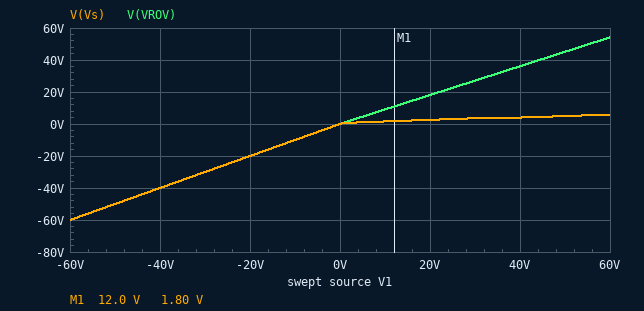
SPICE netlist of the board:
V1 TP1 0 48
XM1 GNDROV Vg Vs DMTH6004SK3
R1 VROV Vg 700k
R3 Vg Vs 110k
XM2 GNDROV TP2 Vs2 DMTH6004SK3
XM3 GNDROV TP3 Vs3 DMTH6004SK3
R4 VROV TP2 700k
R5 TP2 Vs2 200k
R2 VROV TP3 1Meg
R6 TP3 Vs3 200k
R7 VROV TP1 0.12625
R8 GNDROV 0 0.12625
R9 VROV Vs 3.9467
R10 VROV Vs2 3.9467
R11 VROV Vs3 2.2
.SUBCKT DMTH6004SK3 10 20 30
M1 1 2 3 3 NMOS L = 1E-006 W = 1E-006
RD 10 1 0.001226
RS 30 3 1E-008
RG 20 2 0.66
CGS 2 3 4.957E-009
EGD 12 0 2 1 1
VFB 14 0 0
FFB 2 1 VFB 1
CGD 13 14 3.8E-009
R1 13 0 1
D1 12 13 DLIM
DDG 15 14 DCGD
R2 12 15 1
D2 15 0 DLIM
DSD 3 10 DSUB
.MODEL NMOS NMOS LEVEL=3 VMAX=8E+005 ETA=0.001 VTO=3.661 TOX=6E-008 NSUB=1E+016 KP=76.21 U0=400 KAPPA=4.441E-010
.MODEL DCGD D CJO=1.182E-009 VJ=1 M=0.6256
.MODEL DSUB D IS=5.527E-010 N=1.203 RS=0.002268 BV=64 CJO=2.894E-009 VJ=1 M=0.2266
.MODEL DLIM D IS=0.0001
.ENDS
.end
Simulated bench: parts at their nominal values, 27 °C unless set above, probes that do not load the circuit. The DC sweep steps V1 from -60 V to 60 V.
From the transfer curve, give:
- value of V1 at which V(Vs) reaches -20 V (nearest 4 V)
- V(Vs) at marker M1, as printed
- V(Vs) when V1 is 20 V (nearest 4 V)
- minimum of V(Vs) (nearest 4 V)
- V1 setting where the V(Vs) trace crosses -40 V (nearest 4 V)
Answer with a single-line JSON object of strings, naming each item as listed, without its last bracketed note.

{"value of V1 at which V(Vs) reaches -20 V": "-20 V", "V(Vs) at marker M1, as printed": "1.80 V", "V(Vs) when V1 is 20 V": "4 V", "minimum of V(Vs)": "-60 V", "V1 setting where the V(Vs) trace crosses -40 V": "-40 V"}
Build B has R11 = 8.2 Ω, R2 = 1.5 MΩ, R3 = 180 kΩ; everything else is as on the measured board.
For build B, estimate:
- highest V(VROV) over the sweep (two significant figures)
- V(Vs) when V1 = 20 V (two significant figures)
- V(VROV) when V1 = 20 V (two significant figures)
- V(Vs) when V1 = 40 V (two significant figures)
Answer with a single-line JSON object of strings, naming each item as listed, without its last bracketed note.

{"highest V(VROV) over the sweep": "56 V", "V(Vs) when V1 = 20 V": "1.8 V", "V(VROV) when V1 = 20 V": "19 V", "V(Vs) when V1 = 40 V": "2.8 V"}
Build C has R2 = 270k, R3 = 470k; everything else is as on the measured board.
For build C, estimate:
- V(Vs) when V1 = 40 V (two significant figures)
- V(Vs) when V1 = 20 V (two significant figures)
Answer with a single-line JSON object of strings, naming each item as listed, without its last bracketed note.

{"V(Vs) when V1 = 40 V": "3.9 V", "V(Vs) when V1 = 20 V": "2.0 V"}
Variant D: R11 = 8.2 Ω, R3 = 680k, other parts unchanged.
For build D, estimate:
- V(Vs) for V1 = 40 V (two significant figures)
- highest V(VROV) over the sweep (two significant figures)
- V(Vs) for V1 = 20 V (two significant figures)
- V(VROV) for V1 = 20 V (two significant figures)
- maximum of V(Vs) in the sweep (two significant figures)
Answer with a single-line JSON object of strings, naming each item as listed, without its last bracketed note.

{"V(Vs) for V1 = 40 V": "2.8 V", "highest V(VROV) over the sweep": "56 V", "V(Vs) for V1 = 20 V": "1.4 V", "V(VROV) for V1 = 20 V": "19 V", "maximum of V(Vs) in the sweep": "4.1 V"}
